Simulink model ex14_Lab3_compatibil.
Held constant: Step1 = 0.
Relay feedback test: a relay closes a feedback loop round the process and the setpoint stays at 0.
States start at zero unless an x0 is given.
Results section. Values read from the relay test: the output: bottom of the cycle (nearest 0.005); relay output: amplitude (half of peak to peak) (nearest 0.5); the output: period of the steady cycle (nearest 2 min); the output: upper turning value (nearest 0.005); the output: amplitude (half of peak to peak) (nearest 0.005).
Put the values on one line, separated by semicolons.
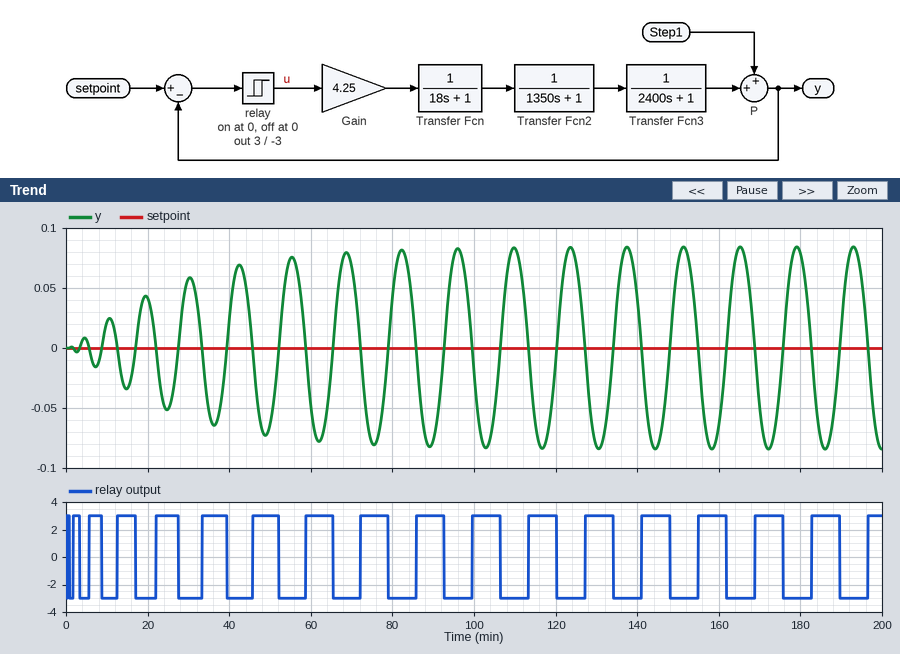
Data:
-0.085; 3.0; 14 min; 0.085; 0.085
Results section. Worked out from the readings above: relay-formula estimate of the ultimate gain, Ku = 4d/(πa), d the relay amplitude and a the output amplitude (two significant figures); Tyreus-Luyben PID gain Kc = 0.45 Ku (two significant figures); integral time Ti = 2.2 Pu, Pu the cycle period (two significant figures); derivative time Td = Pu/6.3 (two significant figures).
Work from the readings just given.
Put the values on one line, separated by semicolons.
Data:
45; 20; 31 min; 2.2 min
